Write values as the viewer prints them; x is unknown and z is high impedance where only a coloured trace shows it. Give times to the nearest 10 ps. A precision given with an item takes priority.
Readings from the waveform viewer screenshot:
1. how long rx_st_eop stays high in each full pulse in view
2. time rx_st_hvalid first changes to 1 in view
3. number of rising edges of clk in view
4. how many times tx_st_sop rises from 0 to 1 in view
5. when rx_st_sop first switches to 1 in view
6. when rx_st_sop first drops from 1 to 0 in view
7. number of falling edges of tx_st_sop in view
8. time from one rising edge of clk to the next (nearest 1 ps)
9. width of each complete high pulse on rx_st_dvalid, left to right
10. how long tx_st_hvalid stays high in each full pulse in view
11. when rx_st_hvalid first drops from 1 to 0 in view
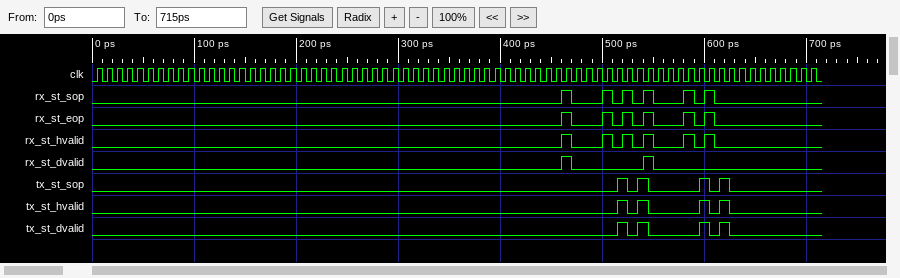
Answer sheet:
10 ps, 10 ps, 10 ps, 10 ps, 10 ps, 10 ps
460 ps
71
4
460 ps
470 ps
4
10 ps
10 ps, 10 ps
10 ps, 10 ps, 10 ps, 10 ps
470 ps
